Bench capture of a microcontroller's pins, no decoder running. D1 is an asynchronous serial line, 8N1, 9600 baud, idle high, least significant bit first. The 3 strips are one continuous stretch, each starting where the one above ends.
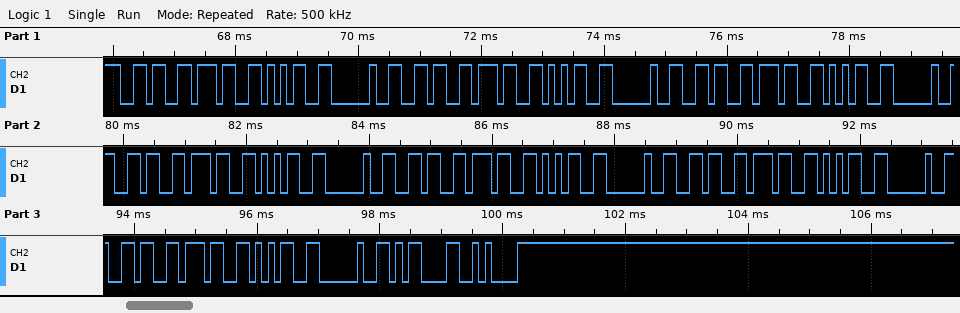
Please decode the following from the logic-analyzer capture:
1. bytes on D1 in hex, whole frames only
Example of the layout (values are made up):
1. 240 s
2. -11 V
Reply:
1. 0x36 0x37 0x35 0x20 0x36 0x37 0x35 0x20 0x36 0x37 0x35 0x20 0x36 0x37 0x35 0x20 0x36 0x37 0x35 0x20 0x36 0x37 0x35 0x20 0x36 0x37 0x35 0x20 0x0D 0x0A
